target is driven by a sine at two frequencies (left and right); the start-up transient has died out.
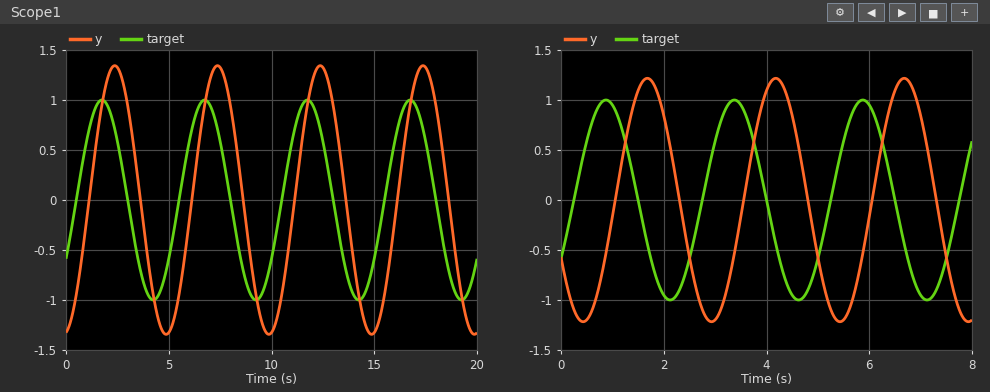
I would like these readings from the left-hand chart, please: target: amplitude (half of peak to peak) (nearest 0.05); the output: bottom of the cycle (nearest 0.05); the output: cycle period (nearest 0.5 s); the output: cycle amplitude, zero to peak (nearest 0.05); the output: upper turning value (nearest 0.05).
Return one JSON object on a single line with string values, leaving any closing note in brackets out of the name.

{"target: amplitude (half of peak to peak)": "1.00", "the output: bottom of the cycle": "-1.35", "the output: cycle period": "5.0 s", "the output: cycle amplitude, zero to peak": "1.35", "the output: upper turning value": "1.35"}
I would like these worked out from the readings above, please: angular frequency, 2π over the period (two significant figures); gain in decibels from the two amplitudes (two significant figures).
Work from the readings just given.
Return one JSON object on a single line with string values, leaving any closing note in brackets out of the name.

{"angular frequency, 2π over the period": "1.3 rad/s", "gain in decibels from the two amplitudes": "2.6 dB"}
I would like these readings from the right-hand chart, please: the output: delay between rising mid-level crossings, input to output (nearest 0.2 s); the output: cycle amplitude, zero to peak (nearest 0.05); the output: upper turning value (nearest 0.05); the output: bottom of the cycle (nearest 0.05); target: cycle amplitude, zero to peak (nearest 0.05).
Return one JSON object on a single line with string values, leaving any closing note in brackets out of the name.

{"the output: delay between rising mid-level crossings, input to output": "0.8 s", "the output: cycle amplitude, zero to peak": "1.20", "the output: upper turning value": "1.20", "the output: bottom of the cycle": "-1.20", "target: cycle amplitude, zero to peak": "1.00"}
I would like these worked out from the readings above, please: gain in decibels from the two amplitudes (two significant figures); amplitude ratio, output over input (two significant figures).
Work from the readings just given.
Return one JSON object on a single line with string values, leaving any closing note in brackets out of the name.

{"gain in decibels from the two amplitudes": "1.6 dB", "amplitude ratio, output over input": "1.2"}
